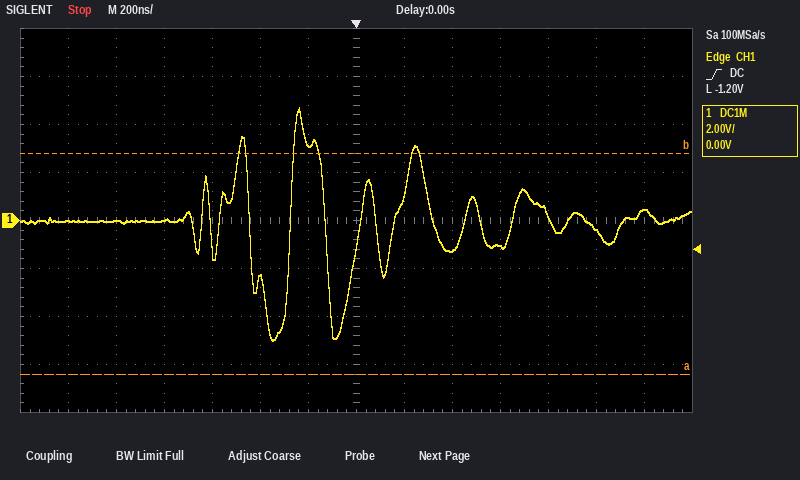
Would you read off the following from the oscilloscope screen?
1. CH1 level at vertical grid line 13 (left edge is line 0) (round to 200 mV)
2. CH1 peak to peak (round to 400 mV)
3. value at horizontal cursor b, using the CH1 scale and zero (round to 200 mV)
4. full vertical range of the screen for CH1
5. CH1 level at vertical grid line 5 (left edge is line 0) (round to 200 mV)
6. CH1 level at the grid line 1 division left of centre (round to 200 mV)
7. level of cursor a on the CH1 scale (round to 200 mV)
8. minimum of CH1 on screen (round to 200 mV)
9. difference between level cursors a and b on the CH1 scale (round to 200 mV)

400 mV
9.6 V
2.8 V
16 V
-2.4 V
3.2 V
-6.4 V
-5.0 V
9.2 V
